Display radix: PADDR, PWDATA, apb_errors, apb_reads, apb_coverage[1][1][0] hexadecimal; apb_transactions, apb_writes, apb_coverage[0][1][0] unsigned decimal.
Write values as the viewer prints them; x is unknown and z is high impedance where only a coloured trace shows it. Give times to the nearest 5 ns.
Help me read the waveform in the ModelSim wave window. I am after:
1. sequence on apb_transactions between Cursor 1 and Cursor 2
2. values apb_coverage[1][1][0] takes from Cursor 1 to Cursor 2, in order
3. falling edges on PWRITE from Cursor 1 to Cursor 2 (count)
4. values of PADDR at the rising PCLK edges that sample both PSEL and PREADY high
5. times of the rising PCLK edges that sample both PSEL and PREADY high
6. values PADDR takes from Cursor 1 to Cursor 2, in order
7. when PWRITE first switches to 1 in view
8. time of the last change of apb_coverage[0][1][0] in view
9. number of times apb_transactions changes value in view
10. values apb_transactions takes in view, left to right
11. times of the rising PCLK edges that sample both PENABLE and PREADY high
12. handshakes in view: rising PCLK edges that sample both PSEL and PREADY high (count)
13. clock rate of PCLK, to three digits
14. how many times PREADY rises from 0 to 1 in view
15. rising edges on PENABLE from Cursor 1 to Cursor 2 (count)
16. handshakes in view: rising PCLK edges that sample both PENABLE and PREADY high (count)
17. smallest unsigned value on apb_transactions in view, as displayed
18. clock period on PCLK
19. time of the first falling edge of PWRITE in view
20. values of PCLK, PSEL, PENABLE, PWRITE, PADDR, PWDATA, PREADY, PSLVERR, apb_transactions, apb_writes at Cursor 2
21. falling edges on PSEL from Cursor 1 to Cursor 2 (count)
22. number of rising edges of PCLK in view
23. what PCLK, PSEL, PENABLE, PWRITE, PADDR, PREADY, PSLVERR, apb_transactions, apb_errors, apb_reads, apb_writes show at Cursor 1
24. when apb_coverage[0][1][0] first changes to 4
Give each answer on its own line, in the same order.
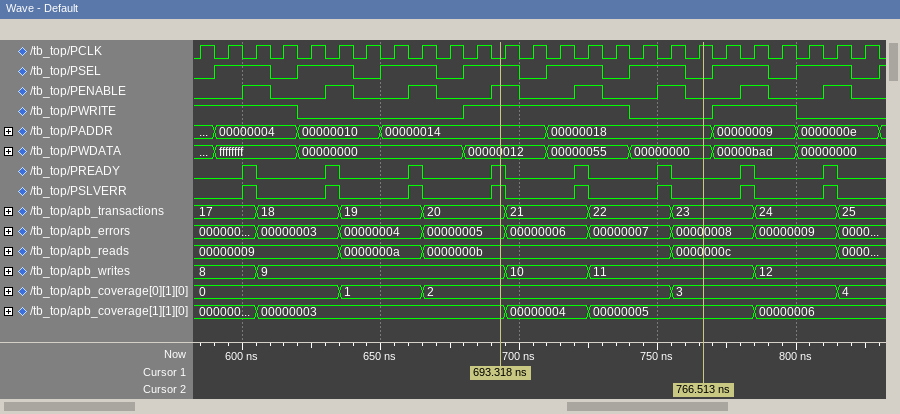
20, 21, 22, 23
00000003, 00000004, 00000005
1
00000004, 00000010, 00000014, 00000014, 00000018, 00000018, 00000009, 0000000e
605 ns, 635 ns, 665 ns, 695 ns, 725 ns, 755 ns, 785 ns, 815 ns
00000014, 00000018
680 ns
815 ns
8
17, 18, 19, 20, 21, 22, 23, 24, 25
605 ns, 635 ns, 665 ns, 695 ns, 725 ns, 755 ns, 785 ns, 815 ns
8
100 MHz
8
2
8
17
10 ns
620 ns
PCLK=1, PSEL=0, PENABLE=0, PWRITE=0, PADDR=00000018, PWDATA=00000000, PREADY=0, PSLVERR=0, apb_transactions=23, apb_writes=11
3
25
PCLK=0, PSEL=1, PENABLE=1, PWRITE=1, PADDR=00000014, PREADY=1, PSLVERR=1, apb_transactions=20, apb_errors=00000005, apb_reads=0000000b, apb_writes=9
815 ns
